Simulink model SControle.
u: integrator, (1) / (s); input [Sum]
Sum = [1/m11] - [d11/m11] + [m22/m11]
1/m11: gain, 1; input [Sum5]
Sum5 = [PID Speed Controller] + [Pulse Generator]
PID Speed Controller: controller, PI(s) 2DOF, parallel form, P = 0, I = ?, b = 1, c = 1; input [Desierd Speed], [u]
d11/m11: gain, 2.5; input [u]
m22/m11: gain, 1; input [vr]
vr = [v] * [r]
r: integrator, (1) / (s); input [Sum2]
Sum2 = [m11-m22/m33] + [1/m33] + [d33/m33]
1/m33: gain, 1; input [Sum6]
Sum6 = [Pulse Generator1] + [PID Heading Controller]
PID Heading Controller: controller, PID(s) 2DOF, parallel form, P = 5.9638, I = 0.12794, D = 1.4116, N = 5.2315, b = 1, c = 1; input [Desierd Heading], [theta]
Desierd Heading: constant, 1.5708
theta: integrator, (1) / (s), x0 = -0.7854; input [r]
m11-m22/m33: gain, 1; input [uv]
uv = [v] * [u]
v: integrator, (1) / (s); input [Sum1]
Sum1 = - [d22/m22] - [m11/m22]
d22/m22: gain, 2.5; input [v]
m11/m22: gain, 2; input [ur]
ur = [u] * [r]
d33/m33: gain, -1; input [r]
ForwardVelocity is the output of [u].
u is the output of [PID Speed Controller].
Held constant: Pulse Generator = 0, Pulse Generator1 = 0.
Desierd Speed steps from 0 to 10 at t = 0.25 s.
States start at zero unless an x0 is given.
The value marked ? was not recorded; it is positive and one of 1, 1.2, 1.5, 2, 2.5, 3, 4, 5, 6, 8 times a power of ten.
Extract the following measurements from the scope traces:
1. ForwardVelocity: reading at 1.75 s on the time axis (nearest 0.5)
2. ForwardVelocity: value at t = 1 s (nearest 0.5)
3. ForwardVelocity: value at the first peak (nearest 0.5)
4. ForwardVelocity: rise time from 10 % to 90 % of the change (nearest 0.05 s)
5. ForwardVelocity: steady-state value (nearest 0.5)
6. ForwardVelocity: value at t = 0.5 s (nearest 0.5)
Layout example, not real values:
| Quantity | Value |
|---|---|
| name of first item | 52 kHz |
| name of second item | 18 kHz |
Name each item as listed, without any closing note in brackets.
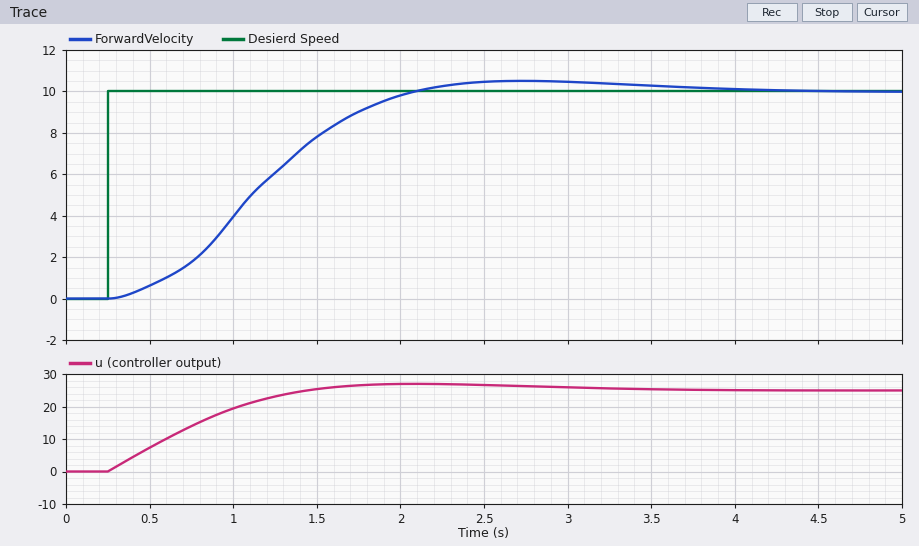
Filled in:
| Quantity | Value |
|---|---|
| ForwardVelocity: reading at 1.75 s on the time axis | 9.0 |
| ForwardVelocity: value at t = 1 s | 4.0 |
| ForwardVelocity: value at the first peak | 10.5 |
| ForwardVelocity: rise time from 10 % to 90 % of the change | 1.15 s |
| ForwardVelocity: steady-state value | 10.0 |
| ForwardVelocity: value at t = 0.5 s | 0.5 |
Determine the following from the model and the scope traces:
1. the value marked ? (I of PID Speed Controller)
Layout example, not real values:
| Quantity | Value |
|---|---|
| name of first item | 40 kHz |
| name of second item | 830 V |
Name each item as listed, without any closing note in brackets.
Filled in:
| Quantity | Value |
|---|---|
| the value marked ? | 3 |
